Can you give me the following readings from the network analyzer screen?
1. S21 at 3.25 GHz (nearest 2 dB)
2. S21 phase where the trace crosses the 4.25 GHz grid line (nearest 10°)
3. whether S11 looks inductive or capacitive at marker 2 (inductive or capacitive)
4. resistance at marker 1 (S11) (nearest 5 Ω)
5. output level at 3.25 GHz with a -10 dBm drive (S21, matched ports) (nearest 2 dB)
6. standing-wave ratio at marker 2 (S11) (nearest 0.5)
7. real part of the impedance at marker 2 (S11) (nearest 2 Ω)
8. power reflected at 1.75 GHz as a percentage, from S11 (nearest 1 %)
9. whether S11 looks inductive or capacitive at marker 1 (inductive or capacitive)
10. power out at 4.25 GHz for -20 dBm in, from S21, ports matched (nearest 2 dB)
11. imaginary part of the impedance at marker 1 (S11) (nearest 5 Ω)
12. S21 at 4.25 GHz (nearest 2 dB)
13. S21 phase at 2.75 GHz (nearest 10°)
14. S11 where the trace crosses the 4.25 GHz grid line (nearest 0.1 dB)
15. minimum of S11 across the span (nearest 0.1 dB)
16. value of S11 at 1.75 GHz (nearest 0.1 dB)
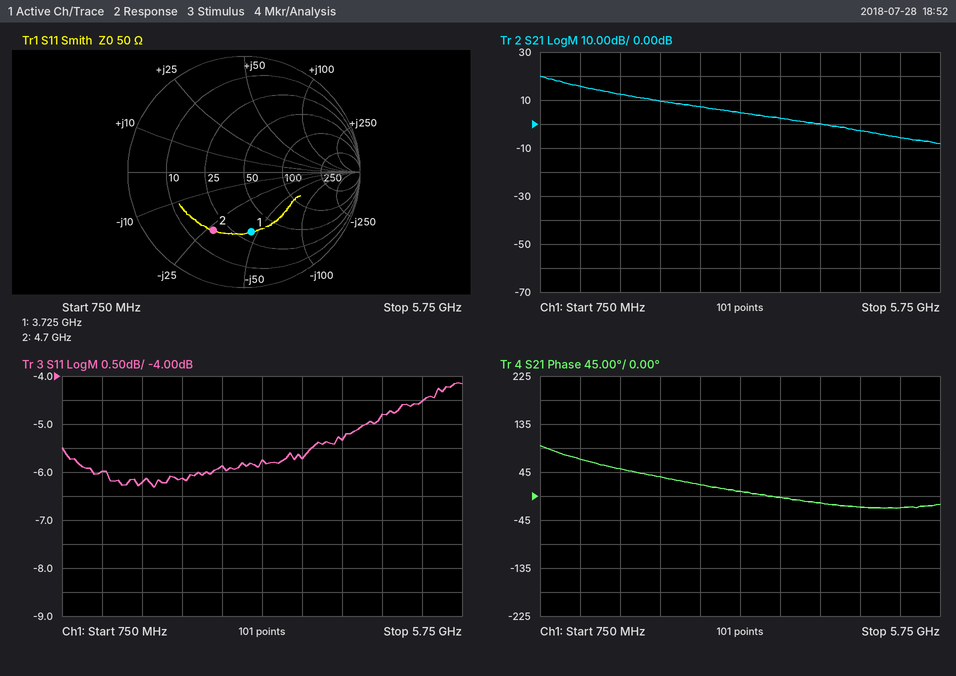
4 dB
-10°
capacitive
30 Ω
-6 dBm
3.5
18 Ω
24 %
capacitive
-20 dBm
-45 Ω
0 dB
20°
-5.3 dB
-6.3 dB
-6.2 dB
